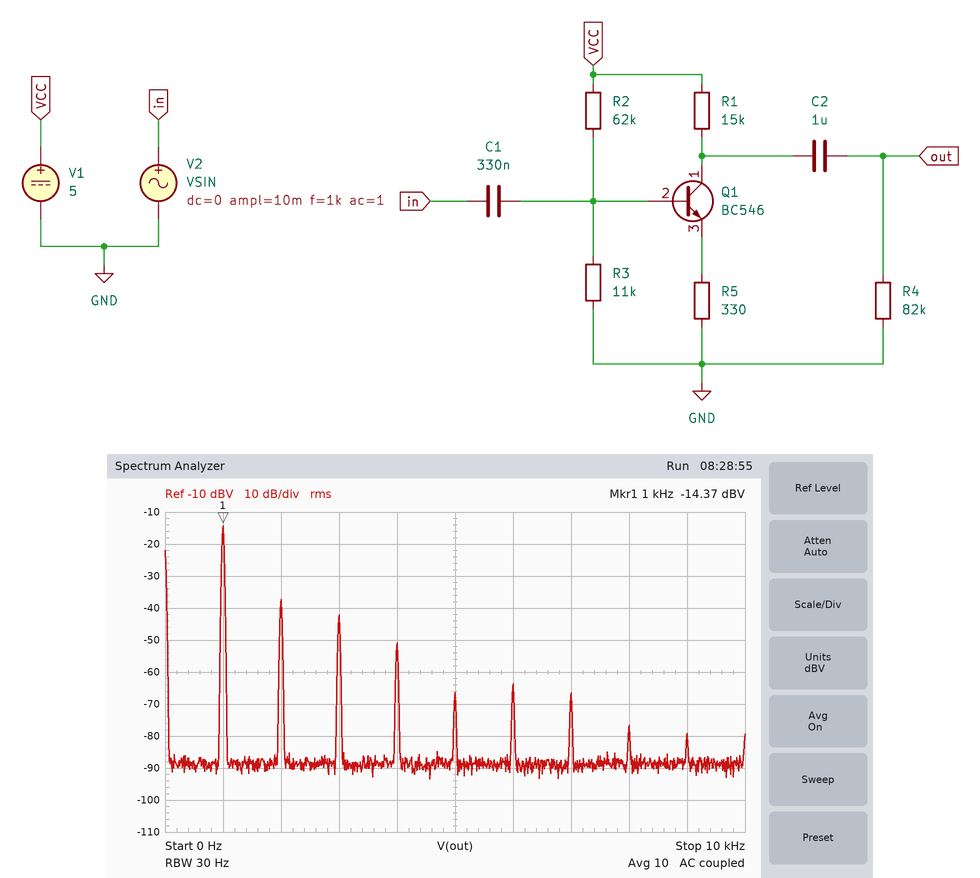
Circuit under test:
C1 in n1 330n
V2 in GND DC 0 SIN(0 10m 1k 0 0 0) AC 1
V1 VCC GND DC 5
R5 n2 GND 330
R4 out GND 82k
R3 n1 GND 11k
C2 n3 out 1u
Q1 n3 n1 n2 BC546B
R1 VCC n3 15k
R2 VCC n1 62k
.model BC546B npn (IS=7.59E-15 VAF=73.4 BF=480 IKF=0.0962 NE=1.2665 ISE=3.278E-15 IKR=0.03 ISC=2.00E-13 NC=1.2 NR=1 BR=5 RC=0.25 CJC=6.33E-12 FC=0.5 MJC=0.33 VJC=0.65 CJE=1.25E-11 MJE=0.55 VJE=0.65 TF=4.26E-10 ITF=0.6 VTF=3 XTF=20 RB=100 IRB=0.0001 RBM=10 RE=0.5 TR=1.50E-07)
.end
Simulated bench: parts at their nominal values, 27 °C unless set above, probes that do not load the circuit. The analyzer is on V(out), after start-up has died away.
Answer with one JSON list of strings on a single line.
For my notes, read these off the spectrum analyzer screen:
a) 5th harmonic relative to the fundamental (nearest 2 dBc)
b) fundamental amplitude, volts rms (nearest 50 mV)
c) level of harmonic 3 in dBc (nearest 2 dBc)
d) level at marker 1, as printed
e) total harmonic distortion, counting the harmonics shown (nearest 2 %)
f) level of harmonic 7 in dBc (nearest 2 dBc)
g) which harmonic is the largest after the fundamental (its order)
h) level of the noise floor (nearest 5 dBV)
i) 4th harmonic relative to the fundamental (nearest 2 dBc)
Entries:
["-52 dBc", "200 mV", "-28 dBc", "-14.37 dBV", "8 %", "-52 dBc", "2", "-90 dBV", "-36 dBc"]
